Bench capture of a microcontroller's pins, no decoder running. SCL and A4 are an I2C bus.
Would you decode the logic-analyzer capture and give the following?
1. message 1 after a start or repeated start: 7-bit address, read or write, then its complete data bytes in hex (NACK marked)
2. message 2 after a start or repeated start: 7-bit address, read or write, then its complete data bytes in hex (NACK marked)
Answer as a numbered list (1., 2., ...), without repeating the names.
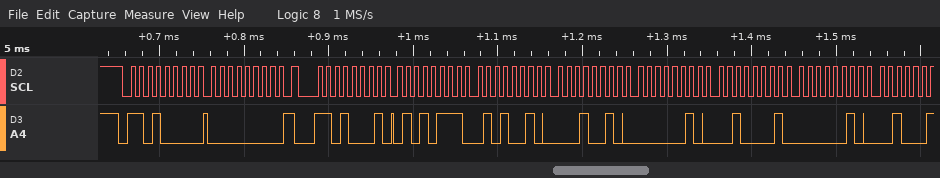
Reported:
1. 0x68 write: 00
2. 0x68 read: 57 52 12 02 21 02
